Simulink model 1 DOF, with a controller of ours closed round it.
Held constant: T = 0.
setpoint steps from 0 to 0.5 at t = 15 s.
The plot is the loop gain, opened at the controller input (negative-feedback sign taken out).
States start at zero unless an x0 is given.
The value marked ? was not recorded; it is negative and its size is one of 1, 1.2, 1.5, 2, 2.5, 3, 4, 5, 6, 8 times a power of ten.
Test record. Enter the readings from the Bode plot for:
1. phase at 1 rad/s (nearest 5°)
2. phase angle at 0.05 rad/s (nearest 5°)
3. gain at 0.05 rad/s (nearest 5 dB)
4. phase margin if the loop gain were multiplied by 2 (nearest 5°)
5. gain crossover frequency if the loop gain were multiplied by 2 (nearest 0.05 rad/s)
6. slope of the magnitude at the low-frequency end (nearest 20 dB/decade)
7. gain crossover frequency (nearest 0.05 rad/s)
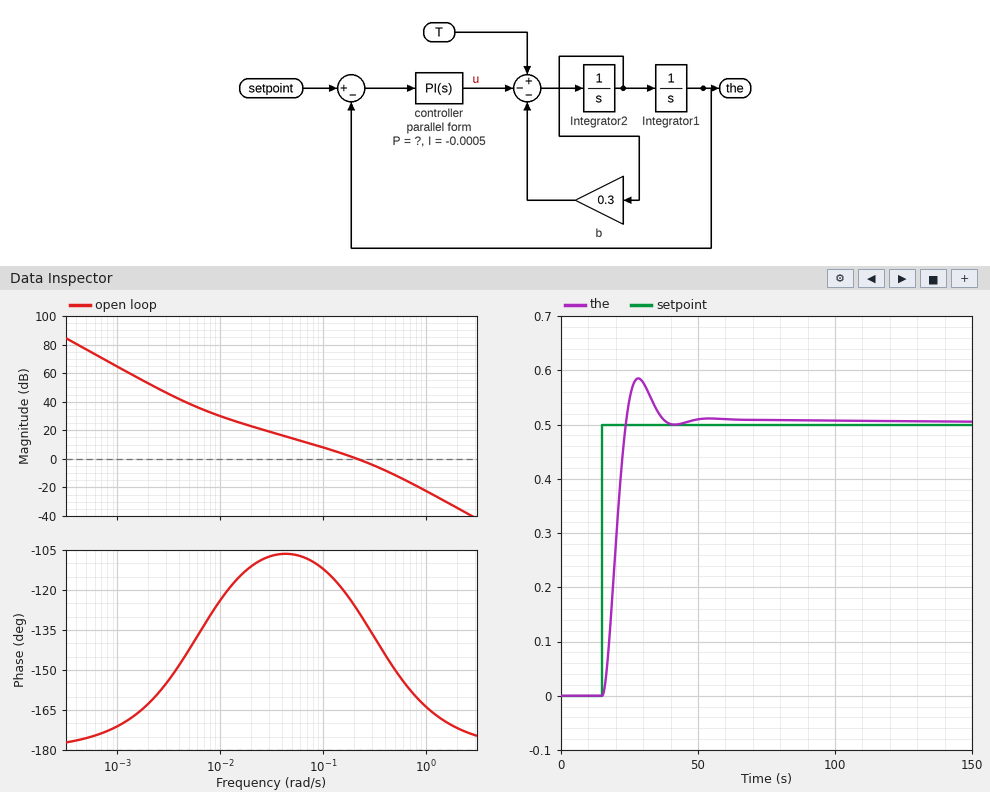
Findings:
-165°
-105°
15 dB
40°
0.35 rad/s
-40 dB/decade
0.20 rad/s
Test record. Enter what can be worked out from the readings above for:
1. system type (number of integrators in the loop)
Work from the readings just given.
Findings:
2
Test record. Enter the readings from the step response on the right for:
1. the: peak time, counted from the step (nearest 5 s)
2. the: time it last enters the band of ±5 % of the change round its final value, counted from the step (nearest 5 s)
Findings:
15 s
20 s
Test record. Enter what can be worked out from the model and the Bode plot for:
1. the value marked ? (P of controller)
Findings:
-0.08
